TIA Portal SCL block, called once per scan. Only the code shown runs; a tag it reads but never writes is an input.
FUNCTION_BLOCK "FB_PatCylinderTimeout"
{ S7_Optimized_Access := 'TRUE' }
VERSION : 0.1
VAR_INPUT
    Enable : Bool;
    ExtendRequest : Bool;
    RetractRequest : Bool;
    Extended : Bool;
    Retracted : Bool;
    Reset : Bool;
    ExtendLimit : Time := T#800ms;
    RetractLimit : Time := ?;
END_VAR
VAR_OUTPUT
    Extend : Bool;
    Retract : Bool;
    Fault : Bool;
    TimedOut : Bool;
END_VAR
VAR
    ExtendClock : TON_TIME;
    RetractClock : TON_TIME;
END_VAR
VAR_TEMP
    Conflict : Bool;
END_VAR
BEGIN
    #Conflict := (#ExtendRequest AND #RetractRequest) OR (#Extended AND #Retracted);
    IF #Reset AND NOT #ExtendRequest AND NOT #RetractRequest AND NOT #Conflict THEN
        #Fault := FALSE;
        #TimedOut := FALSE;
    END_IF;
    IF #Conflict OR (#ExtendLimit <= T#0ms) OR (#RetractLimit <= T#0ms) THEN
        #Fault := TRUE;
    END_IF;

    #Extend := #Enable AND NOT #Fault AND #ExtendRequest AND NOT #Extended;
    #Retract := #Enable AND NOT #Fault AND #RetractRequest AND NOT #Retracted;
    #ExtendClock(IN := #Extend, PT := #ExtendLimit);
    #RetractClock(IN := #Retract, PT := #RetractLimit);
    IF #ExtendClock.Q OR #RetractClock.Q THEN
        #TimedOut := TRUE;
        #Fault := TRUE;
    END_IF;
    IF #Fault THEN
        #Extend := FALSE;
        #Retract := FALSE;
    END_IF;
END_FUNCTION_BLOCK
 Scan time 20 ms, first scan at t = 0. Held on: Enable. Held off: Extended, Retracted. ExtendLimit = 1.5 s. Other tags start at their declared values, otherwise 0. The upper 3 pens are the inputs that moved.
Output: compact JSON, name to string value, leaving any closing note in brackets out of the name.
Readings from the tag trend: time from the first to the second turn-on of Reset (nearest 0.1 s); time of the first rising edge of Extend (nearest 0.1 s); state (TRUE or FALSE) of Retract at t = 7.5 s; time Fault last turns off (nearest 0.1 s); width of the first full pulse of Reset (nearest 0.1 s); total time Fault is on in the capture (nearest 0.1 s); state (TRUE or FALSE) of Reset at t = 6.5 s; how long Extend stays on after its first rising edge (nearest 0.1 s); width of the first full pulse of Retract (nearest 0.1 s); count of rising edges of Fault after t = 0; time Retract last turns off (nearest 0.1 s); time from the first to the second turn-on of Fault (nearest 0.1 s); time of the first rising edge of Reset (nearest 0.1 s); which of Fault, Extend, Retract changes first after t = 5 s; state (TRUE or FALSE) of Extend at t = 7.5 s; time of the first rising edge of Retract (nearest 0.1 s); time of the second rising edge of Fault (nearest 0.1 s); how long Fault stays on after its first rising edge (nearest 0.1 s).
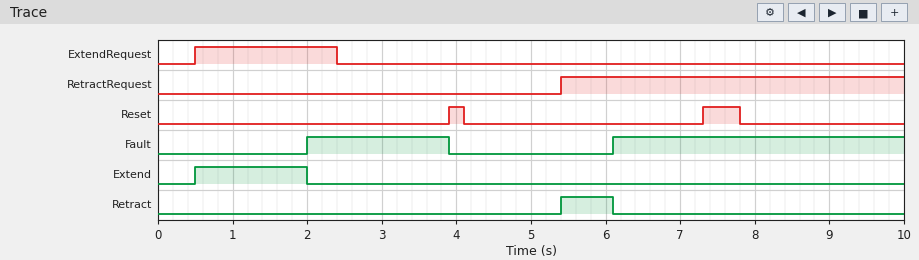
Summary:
{"time from the first to the second turn-on of Reset": "3.4 s", "time of the first rising edge of Extend": "0.5 s", "state (TRUE or FALSE) of Retract at t = 7.5 s": "FALSE", "time Fault last turns off": "3.9 s", "width of the first full pulse of Reset": "0.2 s", "total time Fault is on in the capture": "5.8 s", "state (TRUE or FALSE) of Reset at t = 6.5 s": "FALSE", "how long Extend stays on after its first rising edge": "1.5 s", "width of the first full pulse of Retract": "0.7 s", "count of rising edges of Fault after t = 0": "2", "time Retract last turns off": "6.1 s", "time from the first to the second turn-on of Fault": "4.1 s", "time of the first rising edge of Reset": "3.9 s", "which of Fault, Extend, Retract changes first after t = 5 s": "Retract", "state (TRUE or FALSE) of Extend at t = 7.5 s": "FALSE", "time of the first rising edge of Retract": "5.4 s", "time of the second rising edge of Fault": "6.1 s", "how long Fault stays on after its first rising edge": "1.9 s"}
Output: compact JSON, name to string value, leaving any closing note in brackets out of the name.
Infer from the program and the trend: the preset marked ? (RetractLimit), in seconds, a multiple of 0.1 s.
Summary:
{"the preset marked ? (RetractLimit), in seconds, a multiple of 0.1 s": "0.7 s"}
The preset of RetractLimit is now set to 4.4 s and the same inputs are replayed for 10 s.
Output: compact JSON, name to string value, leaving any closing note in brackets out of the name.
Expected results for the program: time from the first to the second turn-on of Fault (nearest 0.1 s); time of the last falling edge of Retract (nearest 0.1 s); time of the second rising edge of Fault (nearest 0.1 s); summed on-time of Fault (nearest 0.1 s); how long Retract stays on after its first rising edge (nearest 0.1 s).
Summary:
{"time from the first to the second turn-on of Fault": "7.8 s", "time of the last falling edge of Retract": "9.8 s", "time of the second rising edge of Fault": "9.8 s", "summed on-time of Fault": "2.1 s", "how long Retract stays on after its first rising edge": "4.4 s"}
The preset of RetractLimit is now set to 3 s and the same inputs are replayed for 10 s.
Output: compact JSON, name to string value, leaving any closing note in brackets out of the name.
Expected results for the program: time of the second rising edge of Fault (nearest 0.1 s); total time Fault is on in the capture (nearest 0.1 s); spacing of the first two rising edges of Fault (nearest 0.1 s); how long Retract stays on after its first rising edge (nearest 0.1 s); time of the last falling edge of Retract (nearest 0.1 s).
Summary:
{"time of the second rising edge of Fault": "8.4 s", "total time Fault is on in the capture": "3.5 s", "spacing of the first two rising edges of Fault": "6.4 s", "how long Retract stays on after its first rising edge": "3.0 s", "time of the last falling edge of Retract": "8.4 s"}
